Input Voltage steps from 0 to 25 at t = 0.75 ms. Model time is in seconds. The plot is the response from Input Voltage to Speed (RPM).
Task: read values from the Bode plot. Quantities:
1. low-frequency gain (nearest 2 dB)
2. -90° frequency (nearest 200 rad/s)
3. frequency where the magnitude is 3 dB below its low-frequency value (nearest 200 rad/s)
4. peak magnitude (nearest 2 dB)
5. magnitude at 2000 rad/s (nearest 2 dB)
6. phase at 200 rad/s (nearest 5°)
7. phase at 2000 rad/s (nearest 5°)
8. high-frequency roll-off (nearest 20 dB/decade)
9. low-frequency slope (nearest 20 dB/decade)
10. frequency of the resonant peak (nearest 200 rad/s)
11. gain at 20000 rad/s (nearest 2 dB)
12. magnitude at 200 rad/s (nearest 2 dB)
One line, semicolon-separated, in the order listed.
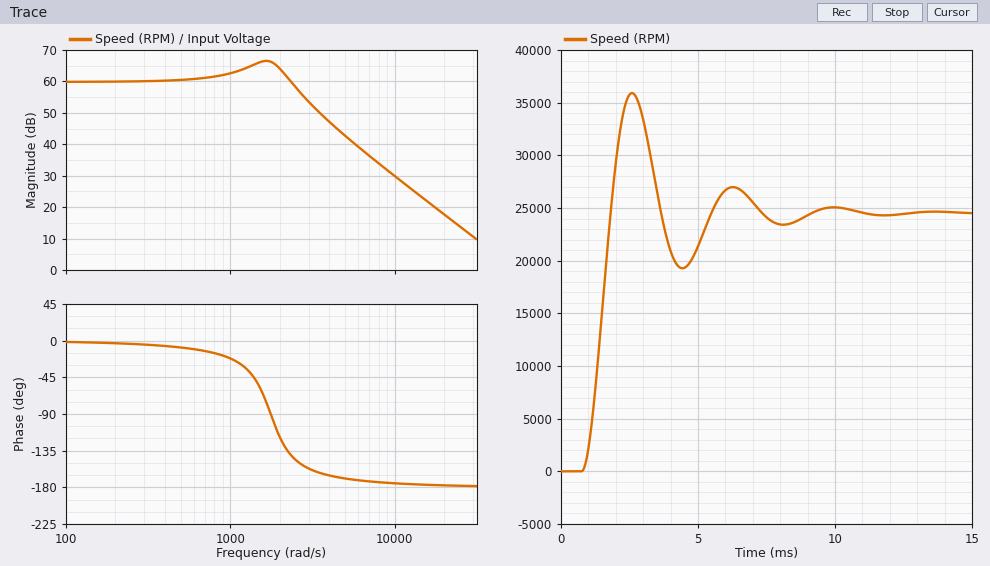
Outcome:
60 dB; 1800 rad/s; 2600 rad/s; 66 dB; 64 dB; -5°; -120°; -40 dB/decade; 0 dB/decade; 1600 rad/s; 18 dB; 60 dB
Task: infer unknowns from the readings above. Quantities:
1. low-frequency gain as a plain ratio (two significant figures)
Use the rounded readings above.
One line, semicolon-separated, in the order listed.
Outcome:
1000
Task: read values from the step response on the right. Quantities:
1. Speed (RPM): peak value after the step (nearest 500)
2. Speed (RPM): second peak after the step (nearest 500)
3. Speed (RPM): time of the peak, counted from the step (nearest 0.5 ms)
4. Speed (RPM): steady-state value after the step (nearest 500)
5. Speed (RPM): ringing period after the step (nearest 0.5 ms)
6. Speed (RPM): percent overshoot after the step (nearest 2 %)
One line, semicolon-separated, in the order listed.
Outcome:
36000; 27000; 2.0 ms; 24500; 3.5 ms; 46 %
